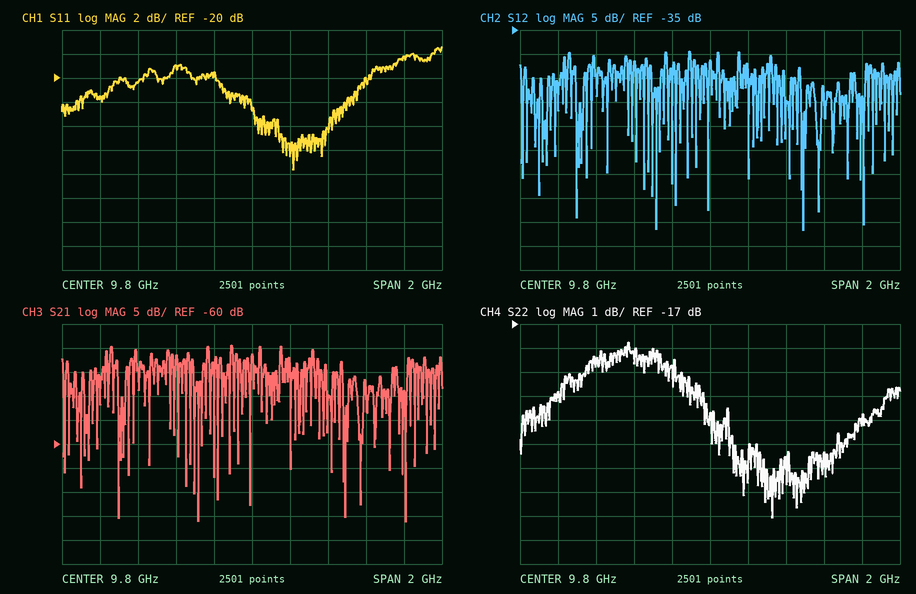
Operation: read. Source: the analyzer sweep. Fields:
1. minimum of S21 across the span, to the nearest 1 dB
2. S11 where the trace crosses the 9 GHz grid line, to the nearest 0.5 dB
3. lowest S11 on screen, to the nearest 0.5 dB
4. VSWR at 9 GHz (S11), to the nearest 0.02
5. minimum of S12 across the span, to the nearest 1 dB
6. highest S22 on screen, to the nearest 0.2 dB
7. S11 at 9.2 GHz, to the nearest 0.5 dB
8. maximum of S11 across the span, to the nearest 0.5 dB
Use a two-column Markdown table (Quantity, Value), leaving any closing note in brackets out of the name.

| Quantity | Value |
|---|---|
| minimum of S21 across the span, to the nearest 1 dB | -76 dB |
| S11 where the trace crosses the 9 GHz grid line, to the nearest 0.5 dB | -21.5 dB |
| lowest S11 on screen, to the nearest 0.5 dB | -27.5 dB |
| VSWR at 9 GHz (S11), to the nearest 0.02 | 1.18 |
| minimum of S12 across the span, to the nearest 1 dB | -77 dB |
| highest S22 on screen, to the nearest 0.2 dB | -17.8 dB |
| S11 at 9.2 GHz, to the nearest 0.5 dB | -20.5 dB |
| maximum of S11 across the span, to the nearest 0.5 dB | -17.5 dB |
